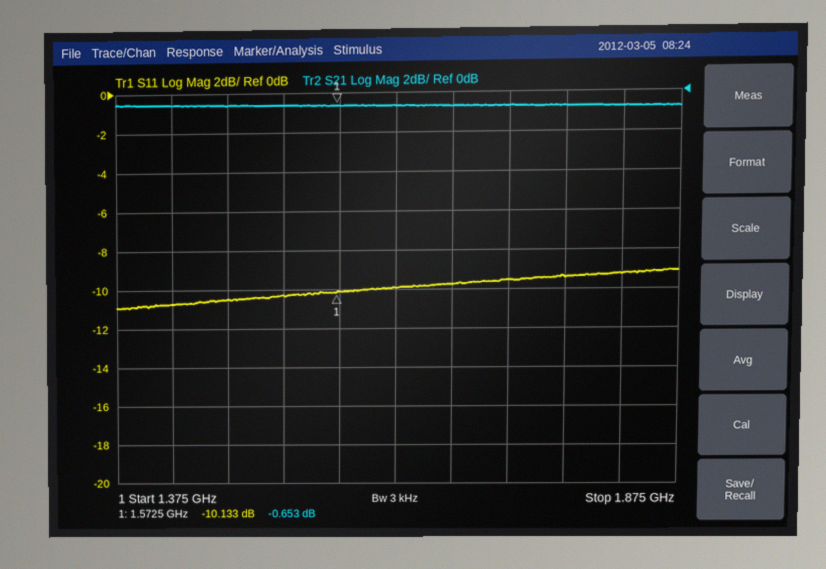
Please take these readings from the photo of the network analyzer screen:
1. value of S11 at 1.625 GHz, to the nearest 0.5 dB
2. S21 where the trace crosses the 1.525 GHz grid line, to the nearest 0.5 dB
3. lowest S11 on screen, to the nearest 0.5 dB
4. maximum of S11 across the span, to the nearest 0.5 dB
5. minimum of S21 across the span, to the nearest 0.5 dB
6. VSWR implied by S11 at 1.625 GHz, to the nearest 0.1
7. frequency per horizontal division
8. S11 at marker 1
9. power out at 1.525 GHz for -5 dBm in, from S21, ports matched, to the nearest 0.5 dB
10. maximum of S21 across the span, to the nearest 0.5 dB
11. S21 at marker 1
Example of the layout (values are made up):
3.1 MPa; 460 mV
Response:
-10.0 dB; -0.5 dB; -11.0 dB; -9.0 dB; -1.0 dB; 1.9; 50 MHz; -10.133 dB; -5.5 dBm; -0.5 dB; -0.653 dB
